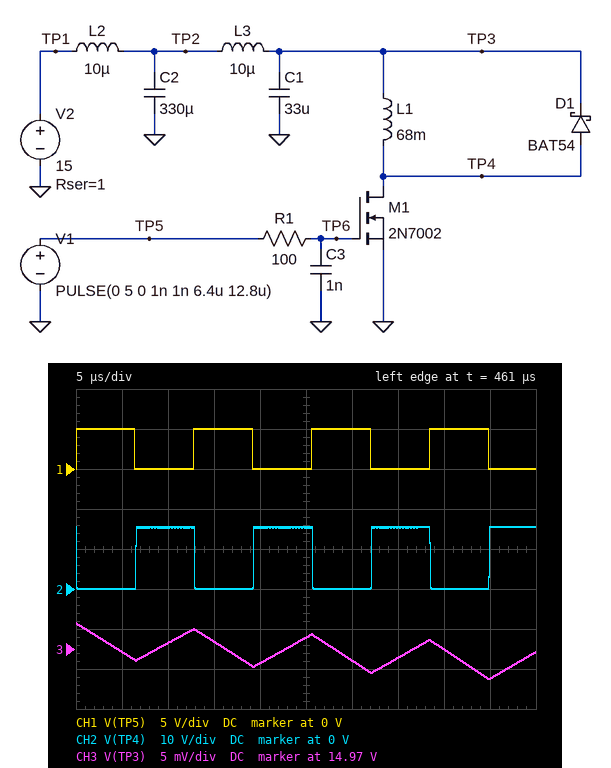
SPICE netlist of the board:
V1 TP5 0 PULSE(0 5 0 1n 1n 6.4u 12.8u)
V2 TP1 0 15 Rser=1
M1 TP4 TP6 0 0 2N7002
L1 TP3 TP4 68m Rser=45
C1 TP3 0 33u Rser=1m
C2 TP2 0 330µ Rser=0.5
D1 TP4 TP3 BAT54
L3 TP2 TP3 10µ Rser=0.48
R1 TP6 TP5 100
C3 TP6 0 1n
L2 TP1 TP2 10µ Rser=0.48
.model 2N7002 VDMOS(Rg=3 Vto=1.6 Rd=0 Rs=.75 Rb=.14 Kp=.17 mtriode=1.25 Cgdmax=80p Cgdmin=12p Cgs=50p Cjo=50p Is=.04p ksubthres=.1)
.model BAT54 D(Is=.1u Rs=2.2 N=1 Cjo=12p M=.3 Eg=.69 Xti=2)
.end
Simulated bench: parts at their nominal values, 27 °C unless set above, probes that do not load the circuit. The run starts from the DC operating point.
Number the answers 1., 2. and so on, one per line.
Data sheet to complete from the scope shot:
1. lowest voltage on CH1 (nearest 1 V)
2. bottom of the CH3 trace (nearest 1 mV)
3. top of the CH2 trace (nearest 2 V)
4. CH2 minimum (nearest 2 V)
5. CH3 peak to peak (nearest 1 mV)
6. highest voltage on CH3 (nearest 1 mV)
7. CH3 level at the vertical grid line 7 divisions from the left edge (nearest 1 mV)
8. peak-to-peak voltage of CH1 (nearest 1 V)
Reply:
1. 0 V
2. 14.971 V
3. 16 V
4. 0 V
5. 7 mV
6. 14.978 V
7. 14.974 V
8. 5 V
